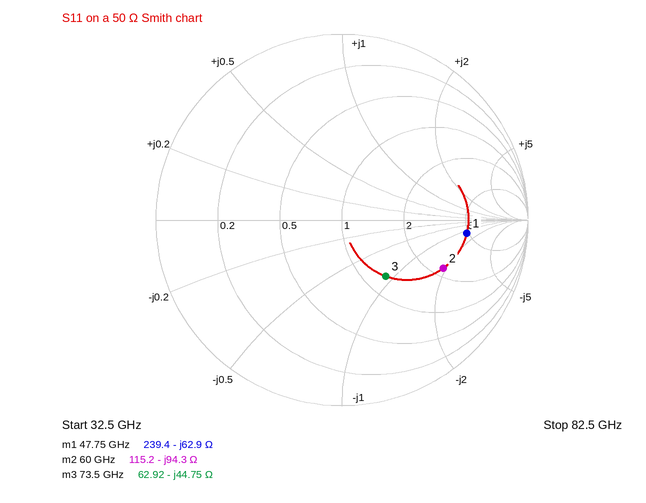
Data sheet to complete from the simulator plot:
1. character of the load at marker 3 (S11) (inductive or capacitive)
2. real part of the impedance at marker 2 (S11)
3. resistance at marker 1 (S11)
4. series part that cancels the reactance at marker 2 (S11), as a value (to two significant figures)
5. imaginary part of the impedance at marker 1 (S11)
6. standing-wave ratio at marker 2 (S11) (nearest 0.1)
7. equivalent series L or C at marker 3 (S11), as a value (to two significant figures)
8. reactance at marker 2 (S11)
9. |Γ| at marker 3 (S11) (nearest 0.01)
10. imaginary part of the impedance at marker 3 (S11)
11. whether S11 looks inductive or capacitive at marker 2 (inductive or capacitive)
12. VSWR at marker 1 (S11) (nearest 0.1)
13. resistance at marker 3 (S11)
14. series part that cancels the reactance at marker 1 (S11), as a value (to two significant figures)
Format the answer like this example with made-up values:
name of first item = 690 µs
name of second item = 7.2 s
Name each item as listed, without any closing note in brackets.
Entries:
character of the load at marker 3 (S11) = capacitive
real part of the impedance at marker 2 = 115.2 Ω
resistance at marker 1 = 239.4 Ω
series part that cancels the reactance at marker 2 (S11), as a value = 250 pH
imaginary part of the impedance at marker 1 = -62.9 Ω
standing-wave ratio at marker 2 (S11) = 4.0
equivalent series L or C at marker 3 (S11), as a value = 48 fF
reactance at marker 2 = -94.3 Ω
|Γ| at marker 3 (S11) = 0.38
imaginary part of the impedance at marker 3 = -44.75 Ω
whether S11 looks inductive or capacitive at marker 2 = capacitive
VSWR at marker 1 (S11) = 5.1
resistance at marker 3 = 62.92 Ω
series part that cancels the reactance at marker 1 (S11), as a value = 210 pH
